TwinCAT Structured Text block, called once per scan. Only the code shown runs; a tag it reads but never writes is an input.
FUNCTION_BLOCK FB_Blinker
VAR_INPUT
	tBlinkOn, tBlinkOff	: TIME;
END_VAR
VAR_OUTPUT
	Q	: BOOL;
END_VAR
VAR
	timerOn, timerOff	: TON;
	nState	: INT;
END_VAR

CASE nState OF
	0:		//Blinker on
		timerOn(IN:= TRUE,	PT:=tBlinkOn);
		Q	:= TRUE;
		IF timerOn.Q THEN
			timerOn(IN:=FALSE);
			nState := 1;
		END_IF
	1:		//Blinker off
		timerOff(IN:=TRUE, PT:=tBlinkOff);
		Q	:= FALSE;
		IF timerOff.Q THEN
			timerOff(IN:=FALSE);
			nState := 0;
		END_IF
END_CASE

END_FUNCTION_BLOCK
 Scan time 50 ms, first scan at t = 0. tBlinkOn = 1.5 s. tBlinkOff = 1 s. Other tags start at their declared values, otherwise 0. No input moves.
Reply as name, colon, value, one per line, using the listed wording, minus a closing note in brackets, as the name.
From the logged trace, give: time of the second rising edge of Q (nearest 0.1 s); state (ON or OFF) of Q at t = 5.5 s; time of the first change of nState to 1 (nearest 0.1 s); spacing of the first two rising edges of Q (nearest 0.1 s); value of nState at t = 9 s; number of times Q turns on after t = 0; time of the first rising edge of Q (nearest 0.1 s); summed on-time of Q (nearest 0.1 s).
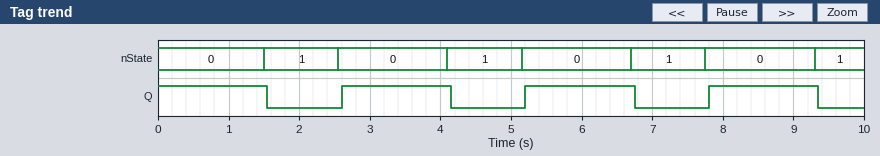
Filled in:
time of the second rising edge of Q: 5.2 s
state (ON or OFF) of Q at t = 5.5 s: ON
time of the first change of nState to 1: 1.5 s
spacing of the first two rising edges of Q: 2.6 s
value of nState at t = 9 s: 0
number of times Q turns on after t = 0: 3
time of the first rising edge of Q: 2.6 s
summed on-time of Q: 6.2 s
